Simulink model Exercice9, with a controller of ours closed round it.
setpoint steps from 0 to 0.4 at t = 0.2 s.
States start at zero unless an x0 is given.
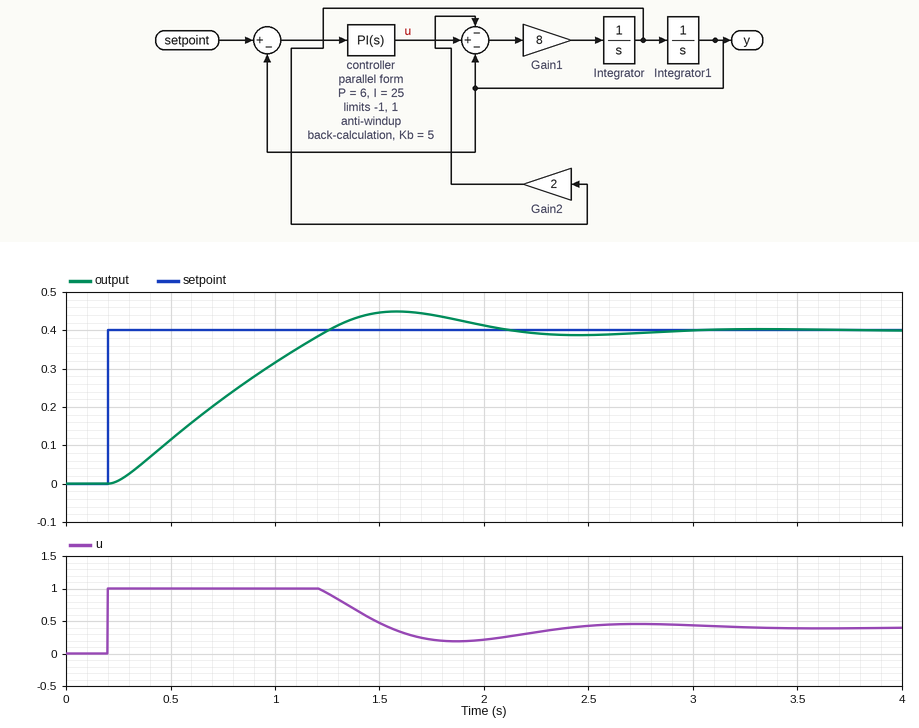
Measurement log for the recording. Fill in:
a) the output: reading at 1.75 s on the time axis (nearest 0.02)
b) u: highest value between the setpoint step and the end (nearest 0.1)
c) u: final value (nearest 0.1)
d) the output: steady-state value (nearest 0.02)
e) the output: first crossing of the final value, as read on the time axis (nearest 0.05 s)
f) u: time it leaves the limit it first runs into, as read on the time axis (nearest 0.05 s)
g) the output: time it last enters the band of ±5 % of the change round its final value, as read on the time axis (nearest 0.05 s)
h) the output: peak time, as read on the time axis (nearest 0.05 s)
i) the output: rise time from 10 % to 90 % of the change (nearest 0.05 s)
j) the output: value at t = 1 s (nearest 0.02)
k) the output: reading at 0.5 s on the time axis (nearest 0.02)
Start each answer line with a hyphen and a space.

- 0.44
- 1.0
- 0.4
- 0.40
- 1.25 s
- 1.20 s
- 1.95 s
- 1.60 s
- 0.80 s
- 0.32
- 0.12
